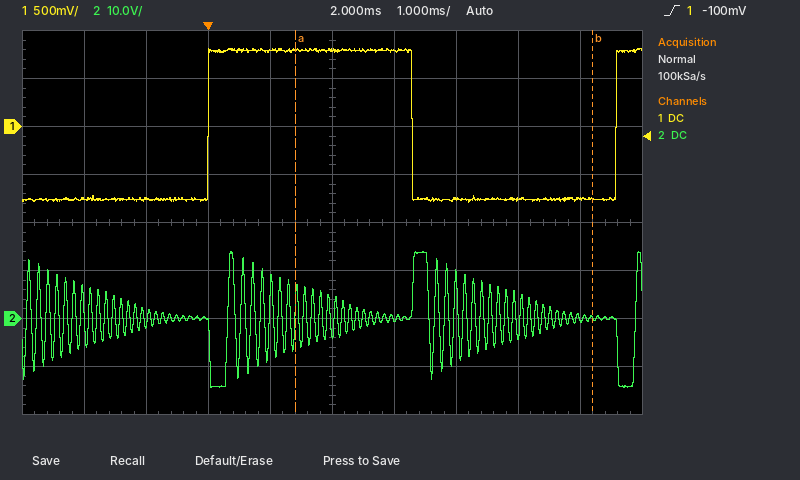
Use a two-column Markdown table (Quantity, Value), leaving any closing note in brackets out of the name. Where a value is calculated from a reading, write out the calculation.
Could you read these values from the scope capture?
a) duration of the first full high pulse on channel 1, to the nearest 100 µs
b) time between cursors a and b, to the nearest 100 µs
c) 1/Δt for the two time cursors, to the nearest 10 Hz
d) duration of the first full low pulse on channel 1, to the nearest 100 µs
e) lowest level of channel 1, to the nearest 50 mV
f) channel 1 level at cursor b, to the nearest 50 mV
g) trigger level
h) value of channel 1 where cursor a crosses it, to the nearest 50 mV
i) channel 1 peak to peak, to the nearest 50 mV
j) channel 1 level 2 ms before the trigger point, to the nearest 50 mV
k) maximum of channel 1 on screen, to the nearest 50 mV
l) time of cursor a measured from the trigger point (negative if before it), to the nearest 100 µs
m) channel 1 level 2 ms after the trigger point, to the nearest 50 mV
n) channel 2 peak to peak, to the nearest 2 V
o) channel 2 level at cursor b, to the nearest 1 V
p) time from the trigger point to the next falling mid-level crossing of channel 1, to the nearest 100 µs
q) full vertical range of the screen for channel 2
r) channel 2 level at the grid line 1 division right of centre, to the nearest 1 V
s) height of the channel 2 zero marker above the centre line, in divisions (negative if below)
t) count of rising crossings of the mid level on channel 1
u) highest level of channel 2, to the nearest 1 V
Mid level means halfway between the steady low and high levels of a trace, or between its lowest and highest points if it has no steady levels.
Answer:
| Quantity | Value |
|---|---|
| duration of the first full high pulse on channel 1, to the nearest 100 µs | 3.3 ms |
| time between cursors a and b, to the nearest 100 µs | 4.8 ms |
| 1/Δt for the two time cursors, to the nearest 10 Hz | 1 / 4.8 ms ≈ 210 Hz |
| duration of the first full low pulse on channel 1, to the nearest 100 µs | 3.3 ms |
| lowest level of channel 1, to the nearest 50 mV | -800 mV |
| channel 1 level at cursor b, to the nearest 50 mV | -750 mV |
| trigger level | -100 mV |
| value of channel 1 where cursor a crosses it, to the nearest 50 mV | 800 mV |
| channel 1 peak to peak, to the nearest 50 mV | 800 mV − (-800 mV) = 1.60 V |
| channel 1 level 2 ms before the trigger point, to the nearest 50 mV | -750 mV |
| maximum of channel 1 on screen, to the nearest 50 mV | 800 mV |
| time of cursor a measured from the trigger point (negative if before it), to the nearest 100 µs | +1.4 ms |
| channel 1 level 2 ms after the trigger point, to the nearest 50 mV | 800 mV |
| channel 2 peak to peak, to the nearest 2 V | 28 V |
| channel 2 level at cursor b, to the nearest 1 V | 0 V |
| time from the trigger point to the next falling mid-level crossing of channel 1, to the nearest 100 µs | 3.3 ms |
| full vertical range of the screen for channel 2 | 80 V |
| channel 2 level at the grid line 1 division right of centre, to the nearest 1 V | 0 V |
| height of the channel 2 zero marker above the centre line, in divisions | -2.0 div |
| count of rising crossings of the mid level on channel 1 | 2 |
| highest level of channel 2, to the nearest 1 V | 14 V |
